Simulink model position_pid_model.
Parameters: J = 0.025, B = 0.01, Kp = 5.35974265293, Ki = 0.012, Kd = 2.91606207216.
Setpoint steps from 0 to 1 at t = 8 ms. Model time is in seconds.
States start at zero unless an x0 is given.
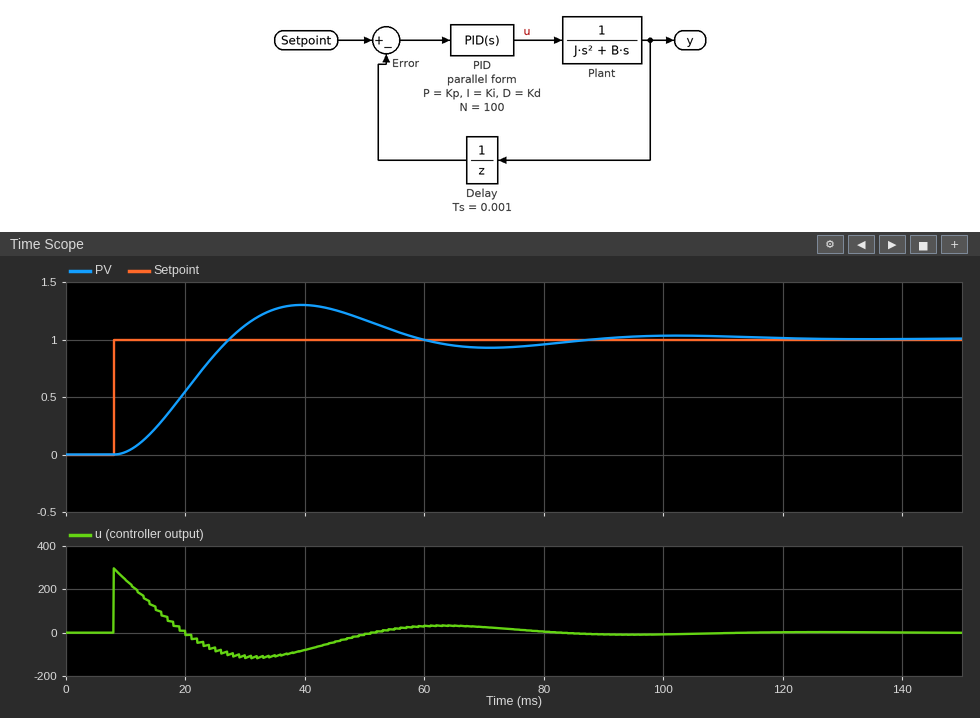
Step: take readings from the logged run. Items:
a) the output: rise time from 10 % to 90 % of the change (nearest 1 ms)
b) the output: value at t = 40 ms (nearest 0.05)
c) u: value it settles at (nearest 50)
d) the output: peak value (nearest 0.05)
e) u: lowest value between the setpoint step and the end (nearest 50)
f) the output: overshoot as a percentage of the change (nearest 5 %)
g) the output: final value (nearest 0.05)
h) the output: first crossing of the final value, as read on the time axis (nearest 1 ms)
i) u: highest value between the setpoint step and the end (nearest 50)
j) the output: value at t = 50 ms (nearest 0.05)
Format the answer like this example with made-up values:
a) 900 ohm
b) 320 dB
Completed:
a) 13 ms
b) 1.30
c) 0
d) 1.30
e) -100
f) 30 %
g) 1.00
h) 27 ms
i) 300
j) 1.15
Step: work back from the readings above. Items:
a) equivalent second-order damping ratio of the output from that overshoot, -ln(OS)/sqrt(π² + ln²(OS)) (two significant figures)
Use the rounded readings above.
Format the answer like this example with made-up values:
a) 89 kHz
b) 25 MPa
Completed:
a) 0.36
